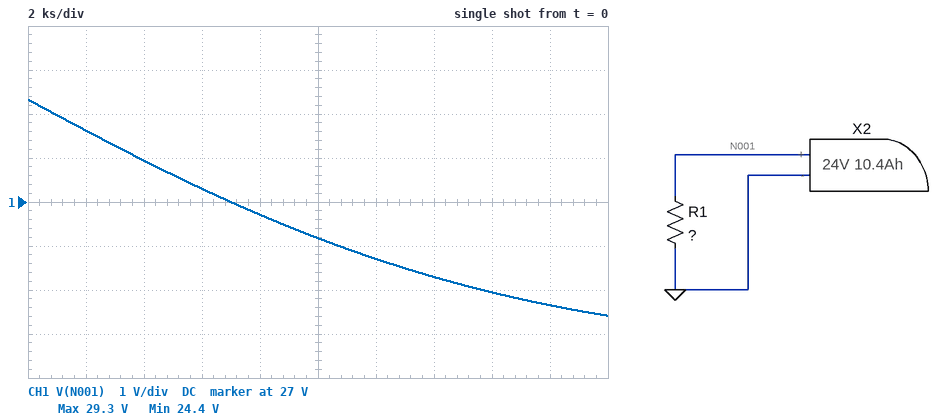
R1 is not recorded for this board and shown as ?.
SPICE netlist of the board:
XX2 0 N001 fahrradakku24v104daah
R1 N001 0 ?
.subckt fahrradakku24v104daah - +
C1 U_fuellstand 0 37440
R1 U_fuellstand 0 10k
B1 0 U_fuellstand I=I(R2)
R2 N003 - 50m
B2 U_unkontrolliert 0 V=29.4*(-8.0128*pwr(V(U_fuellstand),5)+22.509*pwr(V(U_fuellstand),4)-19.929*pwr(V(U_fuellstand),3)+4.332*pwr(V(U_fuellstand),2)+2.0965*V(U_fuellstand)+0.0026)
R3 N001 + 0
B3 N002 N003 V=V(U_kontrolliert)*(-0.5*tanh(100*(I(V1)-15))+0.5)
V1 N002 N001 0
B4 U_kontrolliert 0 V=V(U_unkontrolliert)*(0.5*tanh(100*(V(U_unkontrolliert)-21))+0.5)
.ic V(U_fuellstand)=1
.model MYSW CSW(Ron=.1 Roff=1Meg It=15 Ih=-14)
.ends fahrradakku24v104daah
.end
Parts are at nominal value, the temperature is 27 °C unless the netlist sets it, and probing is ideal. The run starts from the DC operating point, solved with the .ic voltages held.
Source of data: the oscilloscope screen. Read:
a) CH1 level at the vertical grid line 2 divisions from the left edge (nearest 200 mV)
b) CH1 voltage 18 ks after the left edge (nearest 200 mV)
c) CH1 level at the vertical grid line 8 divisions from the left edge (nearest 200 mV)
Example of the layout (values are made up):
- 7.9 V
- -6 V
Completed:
- 28.0 V
- 24.6 V
- 25.0 V
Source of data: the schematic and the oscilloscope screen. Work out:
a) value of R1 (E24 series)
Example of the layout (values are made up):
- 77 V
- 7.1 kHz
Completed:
- 62 Ω
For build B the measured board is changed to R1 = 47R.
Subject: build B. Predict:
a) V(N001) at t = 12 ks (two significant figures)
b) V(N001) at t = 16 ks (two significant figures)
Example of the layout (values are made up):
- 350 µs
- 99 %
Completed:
- 25 V
- 24 V
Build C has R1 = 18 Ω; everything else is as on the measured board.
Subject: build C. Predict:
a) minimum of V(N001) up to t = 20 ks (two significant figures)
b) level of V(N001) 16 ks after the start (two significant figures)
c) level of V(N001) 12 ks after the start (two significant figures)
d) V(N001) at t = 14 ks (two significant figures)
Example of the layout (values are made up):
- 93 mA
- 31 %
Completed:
- 52 mV
- 22 V
- 24 V
- 23 V
